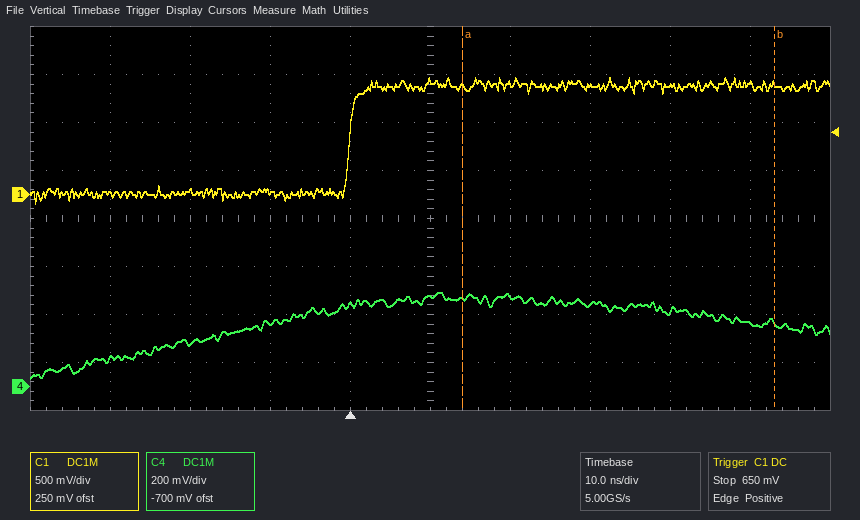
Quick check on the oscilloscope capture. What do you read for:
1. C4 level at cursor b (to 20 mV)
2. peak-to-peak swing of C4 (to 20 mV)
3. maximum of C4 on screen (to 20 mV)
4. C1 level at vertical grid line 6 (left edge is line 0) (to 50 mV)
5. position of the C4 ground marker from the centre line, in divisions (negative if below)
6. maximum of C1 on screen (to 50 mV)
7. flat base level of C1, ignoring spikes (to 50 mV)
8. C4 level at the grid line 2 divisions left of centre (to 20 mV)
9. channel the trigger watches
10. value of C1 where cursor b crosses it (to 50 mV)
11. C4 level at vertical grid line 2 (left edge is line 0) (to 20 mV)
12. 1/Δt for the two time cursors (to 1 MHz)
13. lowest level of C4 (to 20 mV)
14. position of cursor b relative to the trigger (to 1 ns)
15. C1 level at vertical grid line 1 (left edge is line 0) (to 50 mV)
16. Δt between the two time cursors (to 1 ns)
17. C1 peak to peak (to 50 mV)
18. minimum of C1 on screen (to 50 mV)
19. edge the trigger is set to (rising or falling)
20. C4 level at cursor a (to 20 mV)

260 mV
360 mV
400 mV
1.15 V
-3.5 div
1.20 V
0 mV
260 mV
C1
1.15 V
180 mV
26 MHz
40 mV
+53 ns
0 mV
39 ns
1.30 V
-100 mV
rising
360 mV
